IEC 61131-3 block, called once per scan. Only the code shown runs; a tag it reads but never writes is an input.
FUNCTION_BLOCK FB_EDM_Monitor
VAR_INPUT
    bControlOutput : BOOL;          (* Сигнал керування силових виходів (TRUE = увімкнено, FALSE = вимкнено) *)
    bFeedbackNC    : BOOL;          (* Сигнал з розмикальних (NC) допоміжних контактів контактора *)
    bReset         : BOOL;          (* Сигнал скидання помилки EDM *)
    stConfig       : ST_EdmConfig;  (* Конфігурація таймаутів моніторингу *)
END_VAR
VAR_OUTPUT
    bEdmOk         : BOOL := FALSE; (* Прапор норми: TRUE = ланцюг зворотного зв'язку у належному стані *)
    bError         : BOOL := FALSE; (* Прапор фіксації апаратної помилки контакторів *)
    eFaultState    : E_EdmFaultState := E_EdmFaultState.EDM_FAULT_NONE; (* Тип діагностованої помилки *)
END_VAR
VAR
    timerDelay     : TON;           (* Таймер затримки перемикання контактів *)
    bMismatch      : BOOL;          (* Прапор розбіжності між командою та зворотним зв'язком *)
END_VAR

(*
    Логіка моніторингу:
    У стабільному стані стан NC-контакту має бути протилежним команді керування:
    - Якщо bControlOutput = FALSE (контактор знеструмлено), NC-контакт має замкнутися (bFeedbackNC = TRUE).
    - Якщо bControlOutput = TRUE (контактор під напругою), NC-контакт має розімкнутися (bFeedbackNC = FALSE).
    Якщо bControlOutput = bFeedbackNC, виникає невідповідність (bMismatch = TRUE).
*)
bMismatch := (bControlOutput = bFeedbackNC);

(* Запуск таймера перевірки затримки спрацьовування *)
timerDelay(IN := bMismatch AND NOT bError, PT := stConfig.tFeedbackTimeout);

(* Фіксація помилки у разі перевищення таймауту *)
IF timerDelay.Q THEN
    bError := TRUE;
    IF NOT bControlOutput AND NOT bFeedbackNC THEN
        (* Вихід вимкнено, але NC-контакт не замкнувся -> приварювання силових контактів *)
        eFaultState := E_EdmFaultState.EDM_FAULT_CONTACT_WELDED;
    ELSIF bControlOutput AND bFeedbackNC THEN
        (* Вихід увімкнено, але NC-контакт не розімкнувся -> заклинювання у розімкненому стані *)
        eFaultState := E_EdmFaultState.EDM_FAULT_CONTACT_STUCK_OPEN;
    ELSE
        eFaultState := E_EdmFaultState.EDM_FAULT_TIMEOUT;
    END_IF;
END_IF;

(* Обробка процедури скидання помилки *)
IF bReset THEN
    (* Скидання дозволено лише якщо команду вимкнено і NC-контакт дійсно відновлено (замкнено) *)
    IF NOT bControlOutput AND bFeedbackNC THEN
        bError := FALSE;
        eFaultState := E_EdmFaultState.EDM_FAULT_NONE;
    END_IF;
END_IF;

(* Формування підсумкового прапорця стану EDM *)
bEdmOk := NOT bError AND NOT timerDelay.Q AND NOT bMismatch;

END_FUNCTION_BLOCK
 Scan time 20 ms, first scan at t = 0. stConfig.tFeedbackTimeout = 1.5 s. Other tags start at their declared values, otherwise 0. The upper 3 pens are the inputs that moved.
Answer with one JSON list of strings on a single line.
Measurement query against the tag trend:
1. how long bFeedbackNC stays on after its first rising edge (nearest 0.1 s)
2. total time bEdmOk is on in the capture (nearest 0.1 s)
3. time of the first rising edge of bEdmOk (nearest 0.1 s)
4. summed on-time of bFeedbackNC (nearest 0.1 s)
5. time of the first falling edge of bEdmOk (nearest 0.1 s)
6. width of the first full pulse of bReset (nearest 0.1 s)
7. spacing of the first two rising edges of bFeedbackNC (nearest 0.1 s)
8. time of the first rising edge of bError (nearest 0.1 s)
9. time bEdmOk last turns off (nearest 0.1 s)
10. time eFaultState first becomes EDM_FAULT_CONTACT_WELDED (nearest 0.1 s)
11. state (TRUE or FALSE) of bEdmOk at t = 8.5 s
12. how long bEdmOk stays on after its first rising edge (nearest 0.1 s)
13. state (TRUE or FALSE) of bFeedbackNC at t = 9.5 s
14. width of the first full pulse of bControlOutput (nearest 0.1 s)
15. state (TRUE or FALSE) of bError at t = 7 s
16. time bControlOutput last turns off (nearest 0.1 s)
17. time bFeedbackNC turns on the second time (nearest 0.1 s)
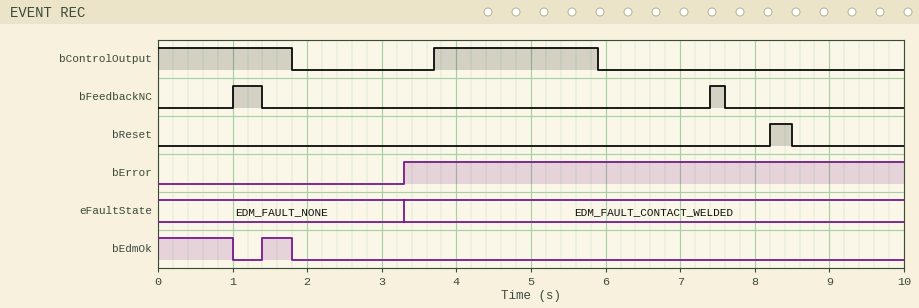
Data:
["0.4 s", "1.4 s", "1.4 s", "0.6 s", "1.0 s", "0.3 s", "6.4 s", "3.3 s", "1.8 s", "3.3 s", "FALSE", "0.4 s", "FALSE", "2.2 s", "TRUE", "5.9 s", "7.4 s"]
